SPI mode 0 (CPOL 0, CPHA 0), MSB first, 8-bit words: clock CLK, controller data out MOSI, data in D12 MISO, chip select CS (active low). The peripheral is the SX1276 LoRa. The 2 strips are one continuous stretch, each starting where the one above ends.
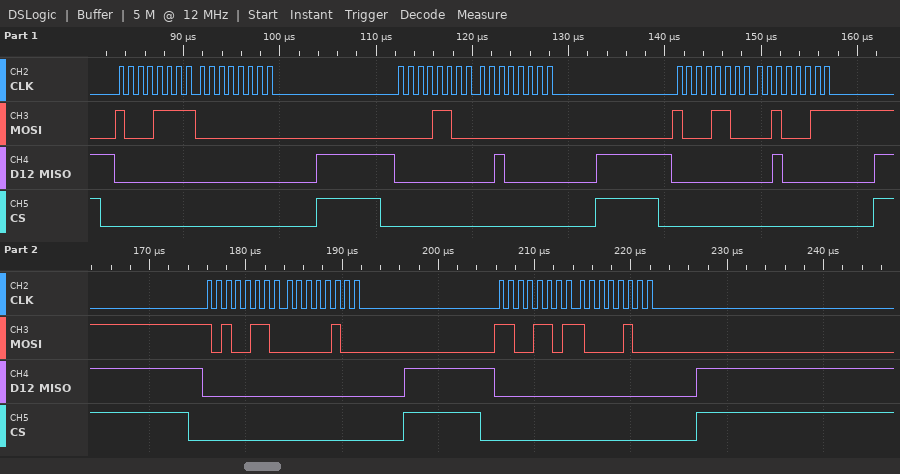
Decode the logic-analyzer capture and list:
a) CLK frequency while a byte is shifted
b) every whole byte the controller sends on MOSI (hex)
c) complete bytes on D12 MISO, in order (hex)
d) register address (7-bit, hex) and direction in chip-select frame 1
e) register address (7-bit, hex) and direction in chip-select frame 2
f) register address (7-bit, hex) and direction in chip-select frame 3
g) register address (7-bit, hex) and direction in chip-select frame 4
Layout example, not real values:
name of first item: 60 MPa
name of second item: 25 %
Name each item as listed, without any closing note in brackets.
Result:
CLK frequency while a byte is shifted: 1 MHz
every whole byte the controller sends on MOSI: 8F 00 0C 00 8C 23 A6 04 CD 84
complete bytes on D12 MISO, in order: 00 00 00 20 00 20 00 00 00 00
register address (7-bit, hex) and direction in chip-select frame 1: 0x0F write
register address (7-bit, hex) and direction in chip-select frame 2: 0x0C read
register address (7-bit, hex) and direction in chip-select frame 3: 0x0C write
register address (7-bit, hex) and direction in chip-select frame 4: 0x26 write
